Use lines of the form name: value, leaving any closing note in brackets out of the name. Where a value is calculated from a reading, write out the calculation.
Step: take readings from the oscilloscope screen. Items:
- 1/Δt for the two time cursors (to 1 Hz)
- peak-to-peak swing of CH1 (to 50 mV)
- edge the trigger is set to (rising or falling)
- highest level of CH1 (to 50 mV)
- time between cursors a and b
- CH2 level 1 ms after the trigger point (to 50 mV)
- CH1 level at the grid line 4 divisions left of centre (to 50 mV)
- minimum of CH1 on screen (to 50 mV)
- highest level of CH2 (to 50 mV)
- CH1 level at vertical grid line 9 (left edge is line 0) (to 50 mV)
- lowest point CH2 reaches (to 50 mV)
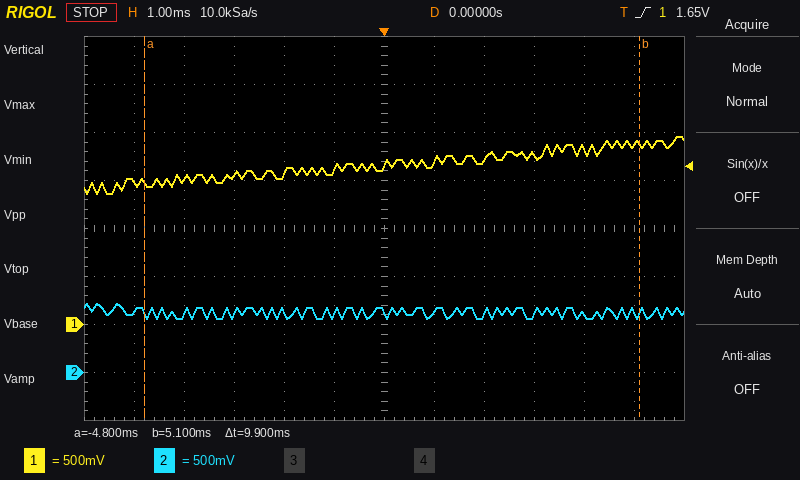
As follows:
1/Δt for the two time cursors: 1 / 9.9 ms ≈ 101 Hz
peak-to-peak swing of CH1: 1.95 V − (1.35 V) = 600 mV
edge the trigger is set to: rising
highest level of CH1: 1.95 V
time between cursors a and b: 9.9 ms
CH2 level 1 ms after the trigger point: 650 mV
CH1 level at the grid line 4 divisions left of centre: 1.50 V
minimum of CH1 on screen: 1.35 V
highest level of CH2: 700 mV
CH1 level at vertical grid line 9 (left edge is line 0): 1.75 V
lowest point CH2 reaches: 550 mV
